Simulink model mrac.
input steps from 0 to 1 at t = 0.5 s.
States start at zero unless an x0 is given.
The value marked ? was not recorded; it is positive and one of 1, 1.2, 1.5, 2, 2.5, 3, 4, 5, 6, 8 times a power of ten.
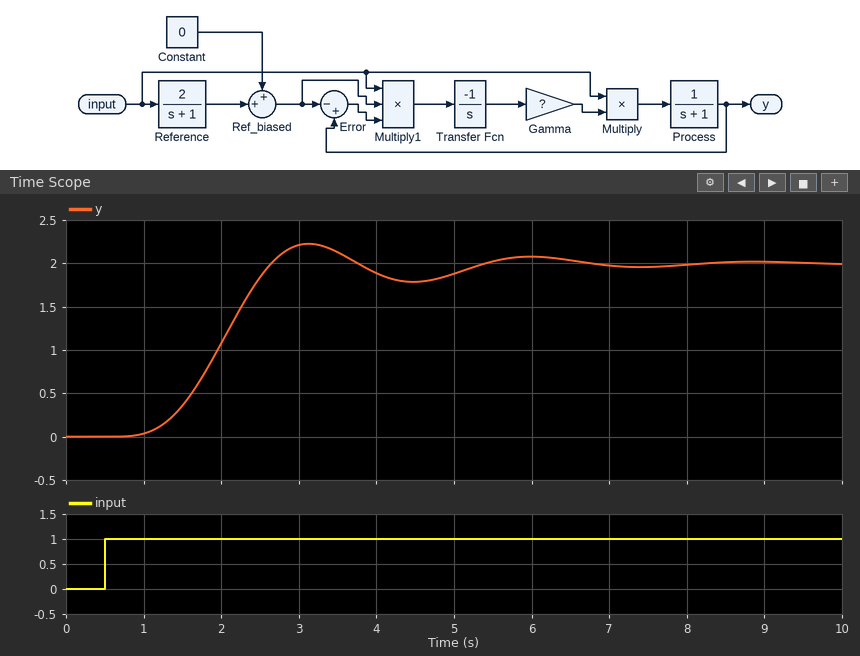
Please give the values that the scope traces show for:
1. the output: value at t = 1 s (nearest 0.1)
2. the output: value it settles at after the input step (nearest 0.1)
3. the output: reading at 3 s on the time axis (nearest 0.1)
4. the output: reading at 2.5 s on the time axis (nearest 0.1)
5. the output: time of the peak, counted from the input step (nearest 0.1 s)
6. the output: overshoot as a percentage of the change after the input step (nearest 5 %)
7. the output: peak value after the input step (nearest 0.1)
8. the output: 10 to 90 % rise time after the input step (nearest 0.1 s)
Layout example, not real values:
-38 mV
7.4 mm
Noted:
0.0
2.0
2.2
1.8
2.6 s
10 %
2.2
1.1 s
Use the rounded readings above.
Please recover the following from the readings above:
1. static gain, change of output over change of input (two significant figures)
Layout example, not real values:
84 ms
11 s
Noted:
2.0
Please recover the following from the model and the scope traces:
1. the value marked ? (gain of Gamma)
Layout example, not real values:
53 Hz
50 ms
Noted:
2.5
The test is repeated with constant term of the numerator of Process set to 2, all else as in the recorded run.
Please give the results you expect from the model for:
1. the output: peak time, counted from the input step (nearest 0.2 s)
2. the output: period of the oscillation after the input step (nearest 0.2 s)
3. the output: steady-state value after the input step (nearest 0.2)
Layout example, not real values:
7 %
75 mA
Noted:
2.0 s
2.0 s
2.0
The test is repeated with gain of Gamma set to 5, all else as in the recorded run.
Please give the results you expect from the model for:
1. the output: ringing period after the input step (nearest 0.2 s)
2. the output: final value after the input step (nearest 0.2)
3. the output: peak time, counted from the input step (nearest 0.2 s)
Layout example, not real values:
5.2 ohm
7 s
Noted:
2.0 s
2.0
2.0 s
